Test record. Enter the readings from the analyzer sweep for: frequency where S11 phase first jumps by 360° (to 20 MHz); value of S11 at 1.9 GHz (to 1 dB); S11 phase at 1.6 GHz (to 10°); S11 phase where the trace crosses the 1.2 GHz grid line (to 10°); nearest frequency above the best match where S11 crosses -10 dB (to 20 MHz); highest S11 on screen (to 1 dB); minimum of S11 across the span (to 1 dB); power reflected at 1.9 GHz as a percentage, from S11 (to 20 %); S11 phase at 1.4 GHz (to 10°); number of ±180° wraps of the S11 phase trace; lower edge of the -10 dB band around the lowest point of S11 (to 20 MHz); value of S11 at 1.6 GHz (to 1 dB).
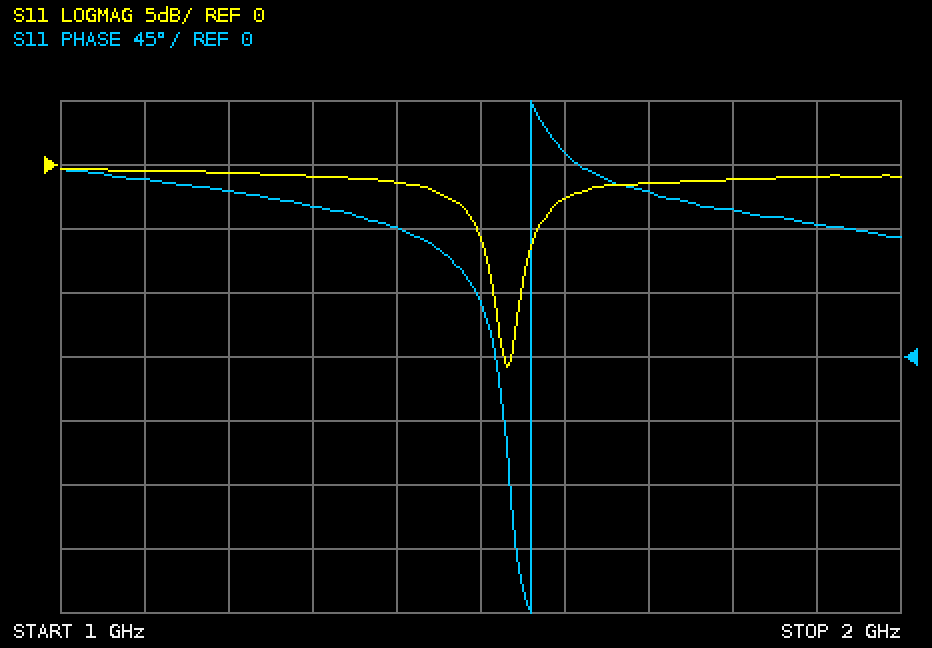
1.56 GHz
-1 dB
140°
120°
1.54 GHz
0 dB
-16 dB
80 %
90°
1
1.52 GHz
-3 dB
